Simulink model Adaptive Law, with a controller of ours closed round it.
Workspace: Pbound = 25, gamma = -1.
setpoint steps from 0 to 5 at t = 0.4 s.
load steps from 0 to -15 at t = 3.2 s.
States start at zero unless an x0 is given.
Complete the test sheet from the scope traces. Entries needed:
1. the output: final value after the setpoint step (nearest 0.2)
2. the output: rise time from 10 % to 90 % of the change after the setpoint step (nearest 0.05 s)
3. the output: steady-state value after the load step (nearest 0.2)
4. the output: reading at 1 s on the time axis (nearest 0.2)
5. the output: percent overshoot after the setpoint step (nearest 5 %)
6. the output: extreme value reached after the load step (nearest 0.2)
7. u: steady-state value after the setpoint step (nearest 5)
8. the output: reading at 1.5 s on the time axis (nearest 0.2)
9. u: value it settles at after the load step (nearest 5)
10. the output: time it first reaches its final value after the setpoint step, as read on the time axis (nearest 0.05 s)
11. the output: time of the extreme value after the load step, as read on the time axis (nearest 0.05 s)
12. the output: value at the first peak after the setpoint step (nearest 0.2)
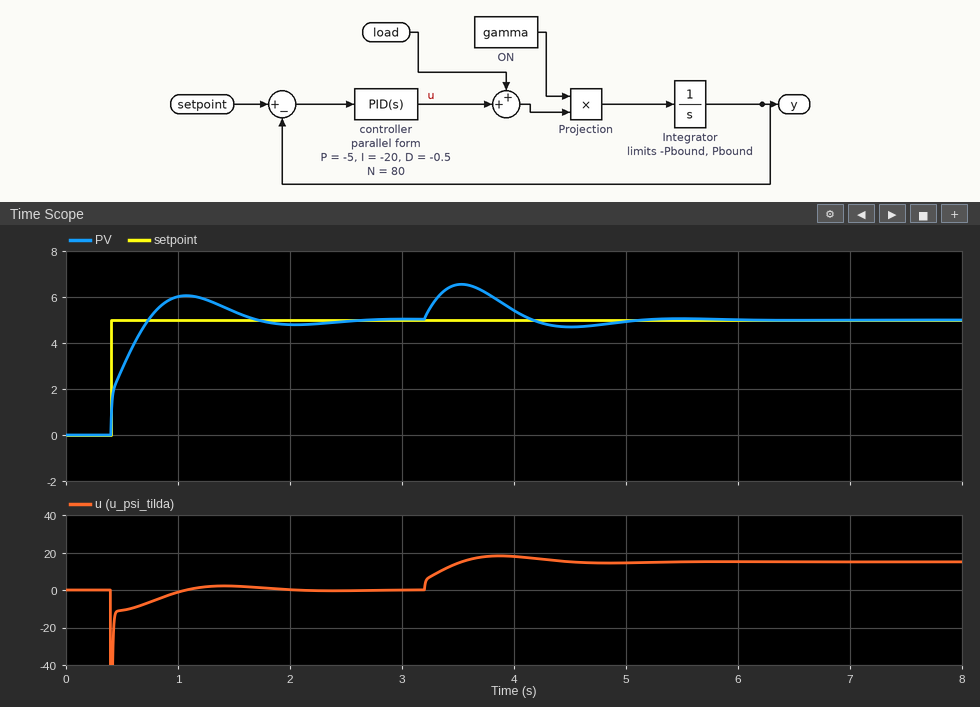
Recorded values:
5.0
0.25 s
5.0
6.0
20 %
6.6
0
5.4
15
0.75 s
3.55 s
6.0
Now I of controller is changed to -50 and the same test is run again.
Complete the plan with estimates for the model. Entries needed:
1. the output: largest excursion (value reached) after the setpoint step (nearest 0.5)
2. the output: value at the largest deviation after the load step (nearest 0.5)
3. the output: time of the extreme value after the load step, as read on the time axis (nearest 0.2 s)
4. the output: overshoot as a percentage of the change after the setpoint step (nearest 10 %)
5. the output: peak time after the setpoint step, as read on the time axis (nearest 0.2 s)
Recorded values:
6.5
6.0
3.4 s
30 %
0.8 s
